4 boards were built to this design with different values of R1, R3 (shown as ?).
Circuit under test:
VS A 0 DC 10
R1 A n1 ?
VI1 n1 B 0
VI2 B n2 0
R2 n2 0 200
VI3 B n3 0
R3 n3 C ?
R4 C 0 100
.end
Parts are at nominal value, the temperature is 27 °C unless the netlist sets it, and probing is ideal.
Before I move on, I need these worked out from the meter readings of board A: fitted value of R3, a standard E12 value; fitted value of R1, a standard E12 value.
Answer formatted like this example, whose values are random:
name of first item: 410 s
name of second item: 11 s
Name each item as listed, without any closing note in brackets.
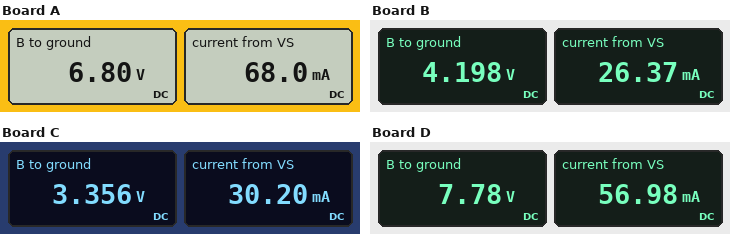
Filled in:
fitted value of R3, a standard E12 value: 100 Ω
fitted value of R1, a standard E12 value: 47 Ω
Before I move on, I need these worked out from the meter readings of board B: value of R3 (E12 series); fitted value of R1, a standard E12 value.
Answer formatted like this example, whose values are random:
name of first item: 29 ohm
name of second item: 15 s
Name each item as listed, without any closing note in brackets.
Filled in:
value of R3: 680 Ω
fitted value of R1, a standard E12 value: 220 Ω
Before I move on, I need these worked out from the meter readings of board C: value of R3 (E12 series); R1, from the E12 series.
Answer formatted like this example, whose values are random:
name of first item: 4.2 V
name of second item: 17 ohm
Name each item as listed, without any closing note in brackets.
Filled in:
value of R3: 150 Ω
R1, from the E12 series: 220 Ω
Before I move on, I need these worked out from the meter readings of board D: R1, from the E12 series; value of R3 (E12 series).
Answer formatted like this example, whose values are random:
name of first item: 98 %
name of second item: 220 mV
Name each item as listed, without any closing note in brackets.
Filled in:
R1, from the E12 series: 39 Ω
value of R3: 330 Ω
